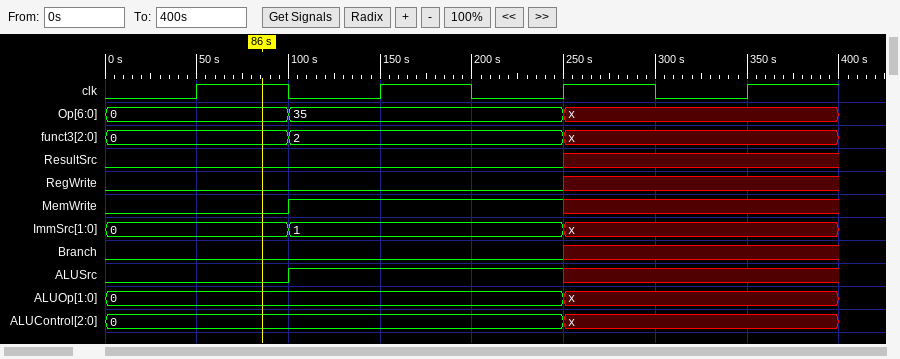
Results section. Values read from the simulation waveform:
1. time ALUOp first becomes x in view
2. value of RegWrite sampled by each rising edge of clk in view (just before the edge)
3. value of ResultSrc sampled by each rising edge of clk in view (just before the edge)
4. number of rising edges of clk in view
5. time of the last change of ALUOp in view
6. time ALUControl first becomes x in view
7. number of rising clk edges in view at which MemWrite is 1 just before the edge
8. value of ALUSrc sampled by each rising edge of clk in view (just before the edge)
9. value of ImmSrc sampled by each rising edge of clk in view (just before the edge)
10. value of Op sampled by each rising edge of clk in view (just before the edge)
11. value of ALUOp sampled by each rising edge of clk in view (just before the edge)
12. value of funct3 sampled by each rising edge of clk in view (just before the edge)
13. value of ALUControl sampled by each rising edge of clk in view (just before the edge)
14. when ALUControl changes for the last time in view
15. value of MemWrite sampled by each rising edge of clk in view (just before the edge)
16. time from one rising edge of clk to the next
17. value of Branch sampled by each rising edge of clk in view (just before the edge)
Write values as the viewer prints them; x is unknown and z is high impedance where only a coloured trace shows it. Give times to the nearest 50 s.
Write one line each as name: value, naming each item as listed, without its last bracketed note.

time ALUOp first becomes x in view: 250 s
value of RegWrite sampled by each rising edge of clk in view: 0 0 0 x
value of ResultSrc sampled by each rising edge of clk in view: 0 0 0 x
number of rising edges of clk in view: 4
time of the last change of ALUOp in view: 250 s
time ALUControl first becomes x in view: 250 s
number of rising clk edges in view at which MemWrite is 1 just before the edge: 2
value of ALUSrc sampled by each rising edge of clk in view: 0 1 1 x
value of ImmSrc sampled by each rising edge of clk in view: 0, 1, 1, x
value of Op sampled by each rising edge of clk in view: 0, 35, 35, x
value of ALUOp sampled by each rising edge of clk in view: 0, 0, 0, x
value of funct3 sampled by each rising edge of clk in view: 0, 2, 2, x
value of ALUControl sampled by each rising edge of clk in view: 0, 0, 0, x
when ALUControl changes for the last time in view: 250 s
value of MemWrite sampled by each rising edge of clk in view: 0 1 1 x
time from one rising edge of clk to the next: 100 s
value of Branch sampled by each rising edge of clk in view: 0 0 0 x
